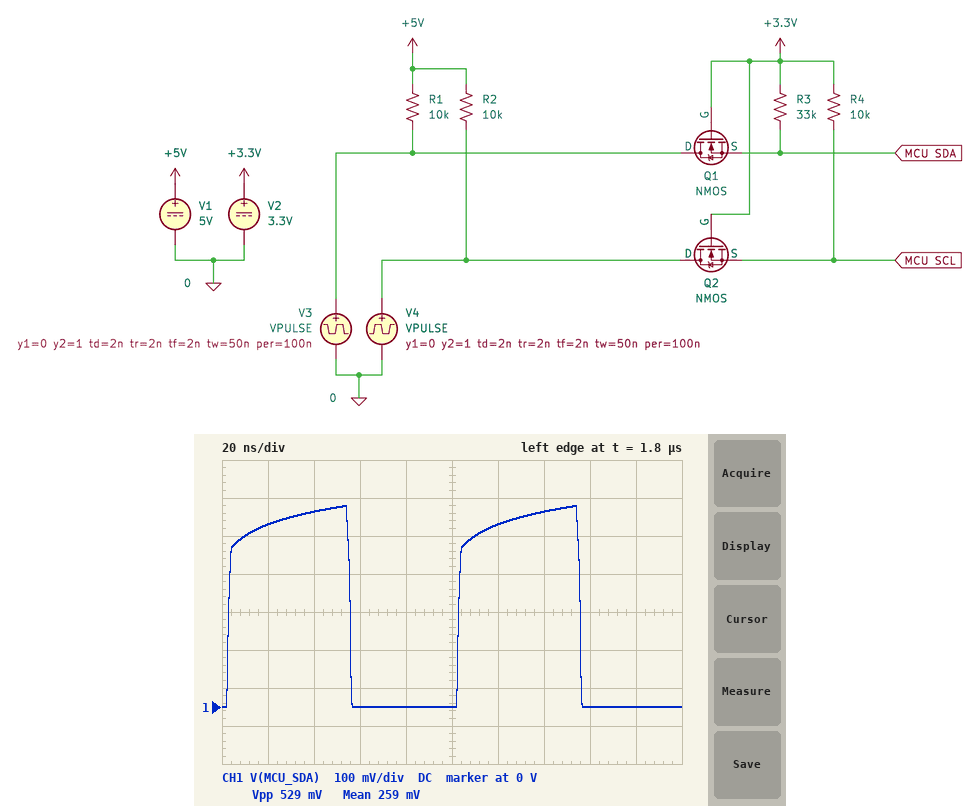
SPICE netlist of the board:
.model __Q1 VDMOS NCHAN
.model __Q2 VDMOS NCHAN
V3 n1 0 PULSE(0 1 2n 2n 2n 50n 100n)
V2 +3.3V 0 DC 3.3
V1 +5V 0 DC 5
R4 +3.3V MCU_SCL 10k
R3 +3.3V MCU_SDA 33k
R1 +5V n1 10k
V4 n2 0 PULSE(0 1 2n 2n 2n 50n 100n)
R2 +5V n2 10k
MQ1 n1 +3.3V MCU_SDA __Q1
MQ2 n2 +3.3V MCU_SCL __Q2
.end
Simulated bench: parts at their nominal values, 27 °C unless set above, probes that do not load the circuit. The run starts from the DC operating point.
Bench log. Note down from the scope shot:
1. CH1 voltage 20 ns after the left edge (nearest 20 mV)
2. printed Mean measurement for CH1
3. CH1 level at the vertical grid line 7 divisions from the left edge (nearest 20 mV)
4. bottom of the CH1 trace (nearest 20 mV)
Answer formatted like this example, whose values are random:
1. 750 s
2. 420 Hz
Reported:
1. 480 mV
2. 259 mV
3. 520 mV
4. 0 V
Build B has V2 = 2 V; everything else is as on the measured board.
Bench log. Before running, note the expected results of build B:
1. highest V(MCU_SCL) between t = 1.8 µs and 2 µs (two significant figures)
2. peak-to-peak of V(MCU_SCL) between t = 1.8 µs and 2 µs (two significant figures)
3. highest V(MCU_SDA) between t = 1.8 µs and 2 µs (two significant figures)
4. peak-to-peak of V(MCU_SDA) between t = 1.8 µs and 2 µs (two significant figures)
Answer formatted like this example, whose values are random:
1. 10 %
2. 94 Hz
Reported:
1. 940 mV
2. 320 mV
3. 890 mV
4. 310 mV
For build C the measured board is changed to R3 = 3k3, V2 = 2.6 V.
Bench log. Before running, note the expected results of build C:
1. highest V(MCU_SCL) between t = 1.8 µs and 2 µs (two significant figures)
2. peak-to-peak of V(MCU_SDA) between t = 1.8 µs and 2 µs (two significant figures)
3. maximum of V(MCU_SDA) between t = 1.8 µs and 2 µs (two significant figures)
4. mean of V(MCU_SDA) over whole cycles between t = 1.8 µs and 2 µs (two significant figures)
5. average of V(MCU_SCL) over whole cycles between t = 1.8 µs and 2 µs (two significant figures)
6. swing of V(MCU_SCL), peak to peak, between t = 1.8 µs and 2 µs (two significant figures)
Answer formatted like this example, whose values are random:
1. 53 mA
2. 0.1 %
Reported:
1. 950 mV
2. 340 mV
3. 990 mV
4. 830 mV
5. 790 mV
6. 320 mV
